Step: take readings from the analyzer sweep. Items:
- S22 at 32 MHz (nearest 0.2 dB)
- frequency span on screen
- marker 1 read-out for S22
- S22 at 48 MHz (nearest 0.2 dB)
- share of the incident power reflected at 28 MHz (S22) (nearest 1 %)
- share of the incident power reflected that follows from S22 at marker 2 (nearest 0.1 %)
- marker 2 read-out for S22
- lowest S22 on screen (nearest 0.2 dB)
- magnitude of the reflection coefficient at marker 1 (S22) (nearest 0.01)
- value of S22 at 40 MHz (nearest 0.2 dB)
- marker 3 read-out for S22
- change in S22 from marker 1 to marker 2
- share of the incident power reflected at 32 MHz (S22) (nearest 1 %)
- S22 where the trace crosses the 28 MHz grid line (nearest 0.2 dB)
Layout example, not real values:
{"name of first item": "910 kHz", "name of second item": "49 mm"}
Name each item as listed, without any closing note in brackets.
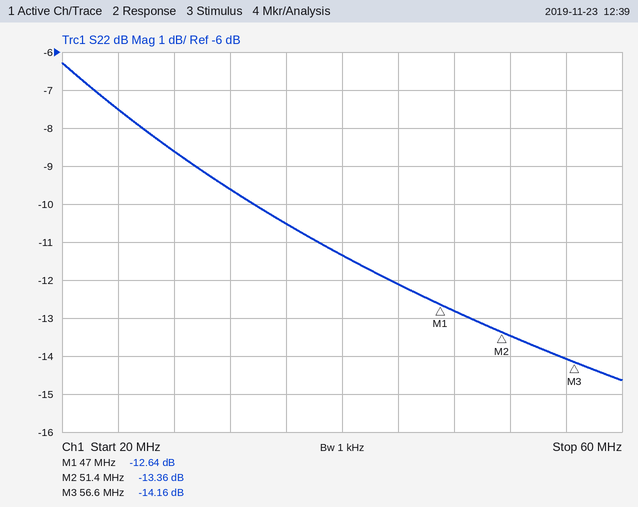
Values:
{"S22 at 32 MHz": "-9.6 dB", "frequency span on screen": "40 MHz", "marker 1 read-out for S22": "-12.64 dB", "S22 at 48 MHz": "-12.8 dB", "share of the incident power reflected at 28 MHz (S22)": "14 %", "share of the incident power reflected that follows from S22 at marker 2": "4.6 %", "marker 2 read-out for S22": "-13.36 dB", "lowest S22 on screen": "-14.6 dB", "magnitude of the reflection coefficient at marker 1 (S22)": "0.23", "value of S22 at 40 MHz": "-11.4 dB", "marker 3 read-out for S22": "-14.16 dB", "change in S22 from marker 1 to marker 2": "-0.72 dB", "share of the incident power reflected at 32 MHz (S22)": "11 %", "S22 where the trace crosses the 28 MHz grid line": "-8.6 dB"}
